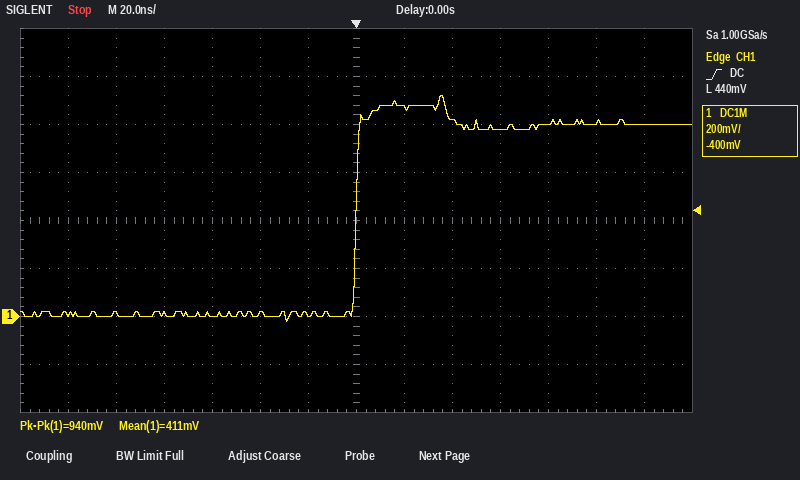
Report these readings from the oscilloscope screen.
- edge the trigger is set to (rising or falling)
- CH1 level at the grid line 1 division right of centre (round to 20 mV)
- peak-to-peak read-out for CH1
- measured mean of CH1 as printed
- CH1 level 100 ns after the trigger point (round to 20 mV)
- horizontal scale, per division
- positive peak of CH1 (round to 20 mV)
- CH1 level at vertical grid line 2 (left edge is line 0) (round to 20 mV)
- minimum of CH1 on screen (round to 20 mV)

rising
880 mV
940 mV
411 mV
800 mV
20 ns
920 mV
20 mV
-20 mV
